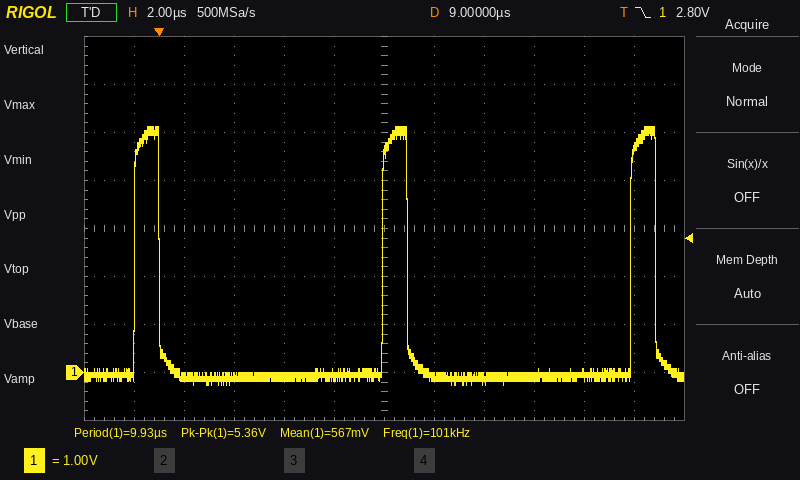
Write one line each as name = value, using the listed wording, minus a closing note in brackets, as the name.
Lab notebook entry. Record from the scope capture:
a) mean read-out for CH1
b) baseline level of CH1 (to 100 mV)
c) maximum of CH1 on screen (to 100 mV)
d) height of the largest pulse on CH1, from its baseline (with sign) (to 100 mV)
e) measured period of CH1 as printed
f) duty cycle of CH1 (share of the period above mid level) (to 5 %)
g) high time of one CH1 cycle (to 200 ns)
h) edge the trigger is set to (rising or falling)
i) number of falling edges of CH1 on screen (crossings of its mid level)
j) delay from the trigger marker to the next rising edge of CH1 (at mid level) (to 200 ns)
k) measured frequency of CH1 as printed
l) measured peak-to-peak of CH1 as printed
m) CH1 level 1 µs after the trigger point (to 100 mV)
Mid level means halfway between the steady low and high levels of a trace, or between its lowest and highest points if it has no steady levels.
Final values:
mean read-out for CH1 = 567 mV
baseline level of CH1 = -100 mV
maximum of CH1 on screen = 5.1 V
height of the largest pulse on CH1, from its baseline (with sign) = +5.2 V
measured period of CH1 as printed = 9.93 µs
duty cycle of CH1 (share of the period above mid level) = 10 %
high time of one CH1 cycle = 1.0 µs
edge the trigger is set to = falling
number of falling edges of CH1 on screen = 3
delay from the trigger marker to the next rising edge of CH1 (at mid level) = 9.0 µs
measured frequency of CH1 as printed = 101 kHz
measured peak-to-peak of CH1 as printed = 5.36 V
CH1 level 1 µs after the trigger point = -100 mV
